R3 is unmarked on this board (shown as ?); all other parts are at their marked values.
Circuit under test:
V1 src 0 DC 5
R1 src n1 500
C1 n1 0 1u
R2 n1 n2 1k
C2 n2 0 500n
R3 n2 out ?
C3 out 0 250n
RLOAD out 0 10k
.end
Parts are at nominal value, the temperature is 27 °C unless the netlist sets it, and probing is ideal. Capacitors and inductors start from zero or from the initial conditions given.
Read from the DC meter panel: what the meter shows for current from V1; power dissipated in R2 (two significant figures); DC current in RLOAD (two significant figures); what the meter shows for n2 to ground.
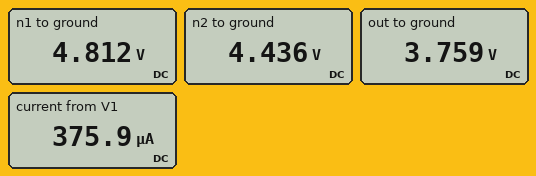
375.9 µA
140 µW
380 µA
4.436 V
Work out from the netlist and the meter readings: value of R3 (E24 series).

1.8 kΩ
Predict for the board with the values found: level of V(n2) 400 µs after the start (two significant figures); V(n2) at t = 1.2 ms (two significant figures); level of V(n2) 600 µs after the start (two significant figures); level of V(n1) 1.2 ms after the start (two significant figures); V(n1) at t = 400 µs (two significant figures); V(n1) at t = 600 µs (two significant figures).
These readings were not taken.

780 mV
2.5 V
1.3 V
3.9 V
2.4 V
3.0 V
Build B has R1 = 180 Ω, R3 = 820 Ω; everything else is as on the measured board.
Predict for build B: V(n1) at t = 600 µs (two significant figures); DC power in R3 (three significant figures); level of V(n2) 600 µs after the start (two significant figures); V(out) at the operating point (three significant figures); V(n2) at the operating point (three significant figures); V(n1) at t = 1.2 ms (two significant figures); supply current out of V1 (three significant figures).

4.4 V
142 µW
2.0 V
4.17 V
4.51 V
4.7 V
417 µA
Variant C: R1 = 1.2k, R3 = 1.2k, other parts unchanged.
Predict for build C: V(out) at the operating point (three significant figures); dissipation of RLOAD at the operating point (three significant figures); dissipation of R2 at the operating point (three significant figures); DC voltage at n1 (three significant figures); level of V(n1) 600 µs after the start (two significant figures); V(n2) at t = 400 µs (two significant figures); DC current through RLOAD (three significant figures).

3.73 V
1.39 mW
139 µW
4.55 V
1.6 V
360 mV
373 µA
